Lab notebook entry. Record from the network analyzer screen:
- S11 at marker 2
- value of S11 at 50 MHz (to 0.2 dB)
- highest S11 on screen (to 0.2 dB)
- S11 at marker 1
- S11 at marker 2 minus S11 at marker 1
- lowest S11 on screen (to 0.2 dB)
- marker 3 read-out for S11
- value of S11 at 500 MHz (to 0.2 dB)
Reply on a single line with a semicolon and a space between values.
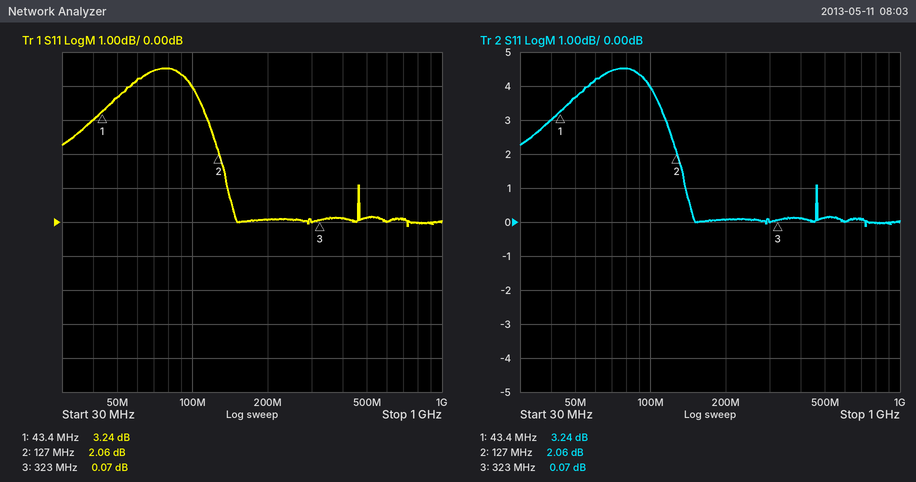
2.06 dB; 3.6 dB; 4.6 dB; 3.24 dB; -1.18 dB; -0.2 dB; 0.07 dB; 0.2 dB
